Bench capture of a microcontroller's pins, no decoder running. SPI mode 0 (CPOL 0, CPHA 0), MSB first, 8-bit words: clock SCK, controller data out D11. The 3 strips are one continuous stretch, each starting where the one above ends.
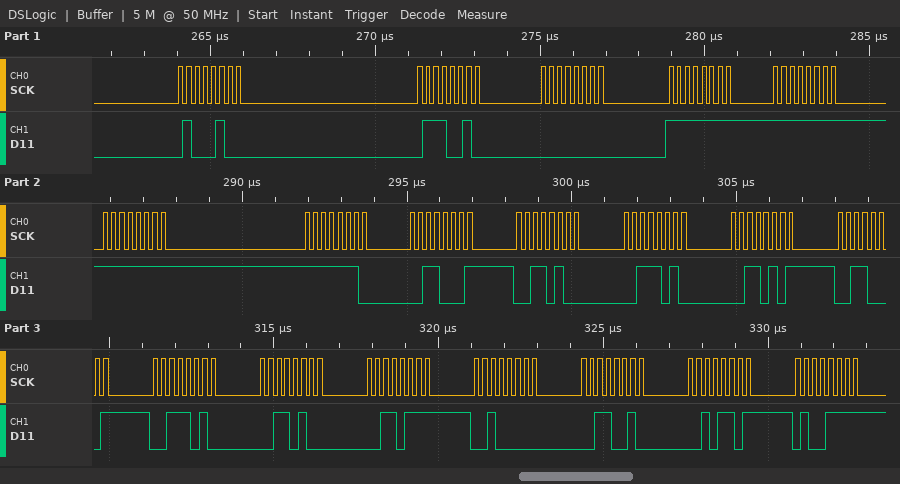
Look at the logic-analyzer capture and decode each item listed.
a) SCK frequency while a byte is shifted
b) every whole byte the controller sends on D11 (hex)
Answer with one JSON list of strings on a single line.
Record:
["4 MHz", "44 72 00 FF FF FF FE 31 34 3A 35 31 3A 34 37 20 32 2D 4F"]
